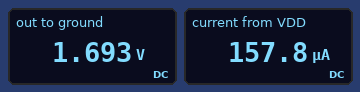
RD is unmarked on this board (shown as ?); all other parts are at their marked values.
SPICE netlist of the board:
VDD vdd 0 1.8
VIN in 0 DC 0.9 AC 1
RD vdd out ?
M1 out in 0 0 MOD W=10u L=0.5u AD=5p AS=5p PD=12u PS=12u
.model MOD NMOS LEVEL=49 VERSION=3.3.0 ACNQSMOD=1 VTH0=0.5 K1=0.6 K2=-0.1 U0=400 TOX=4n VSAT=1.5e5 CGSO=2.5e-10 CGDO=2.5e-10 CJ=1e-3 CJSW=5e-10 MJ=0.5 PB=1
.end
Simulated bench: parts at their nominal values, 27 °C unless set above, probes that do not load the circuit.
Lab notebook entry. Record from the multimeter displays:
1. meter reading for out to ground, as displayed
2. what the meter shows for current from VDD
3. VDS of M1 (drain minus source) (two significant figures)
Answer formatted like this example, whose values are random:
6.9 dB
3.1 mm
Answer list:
1.693 V
157.8 µA
1.7 V
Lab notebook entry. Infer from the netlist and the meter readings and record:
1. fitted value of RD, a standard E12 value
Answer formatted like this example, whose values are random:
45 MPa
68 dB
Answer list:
680 Ω
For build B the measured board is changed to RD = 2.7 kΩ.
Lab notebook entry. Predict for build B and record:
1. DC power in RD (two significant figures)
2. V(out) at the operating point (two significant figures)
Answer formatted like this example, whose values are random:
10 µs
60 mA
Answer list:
65 µW
1.4 V
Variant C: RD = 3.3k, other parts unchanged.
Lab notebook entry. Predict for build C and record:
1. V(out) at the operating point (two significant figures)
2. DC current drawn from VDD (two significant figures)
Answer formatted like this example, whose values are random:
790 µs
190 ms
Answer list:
1.3 V
150 µA
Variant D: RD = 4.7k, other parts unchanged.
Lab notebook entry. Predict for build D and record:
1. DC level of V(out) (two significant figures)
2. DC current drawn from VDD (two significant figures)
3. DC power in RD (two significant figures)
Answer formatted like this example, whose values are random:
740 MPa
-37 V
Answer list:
1.1 V
150 µA
110 µW
